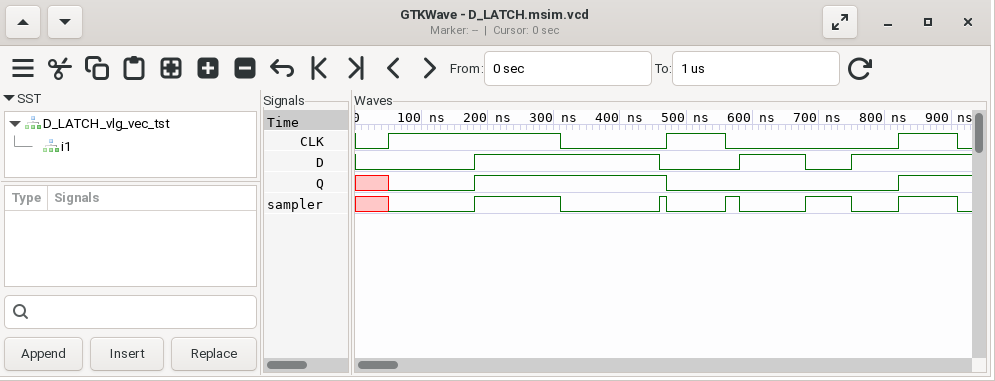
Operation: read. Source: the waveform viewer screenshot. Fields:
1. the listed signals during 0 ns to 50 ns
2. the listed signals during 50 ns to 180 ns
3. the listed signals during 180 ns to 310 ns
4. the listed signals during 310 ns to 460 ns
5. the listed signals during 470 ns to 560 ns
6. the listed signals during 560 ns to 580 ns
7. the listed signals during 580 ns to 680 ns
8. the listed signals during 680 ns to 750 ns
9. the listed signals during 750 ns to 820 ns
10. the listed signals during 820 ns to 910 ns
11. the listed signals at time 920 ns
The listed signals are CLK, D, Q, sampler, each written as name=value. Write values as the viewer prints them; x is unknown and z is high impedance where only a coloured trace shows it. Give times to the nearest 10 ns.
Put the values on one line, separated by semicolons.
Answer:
CLK=0, D=0, Q=x, sampler=x; CLK=1, D=0, Q=0, sampler=0; CLK=1, D=1, Q=1, sampler=1; CLK=0, D=1, Q=1, sampler=0; CLK=1, D=0, Q=0, sampler=0; CLK=0, D=0, Q=0, sampler=1; CLK=0, D=1, Q=0, sampler=0; CLK=0, D=0, Q=0, sampler=1; CLK=0, D=1, Q=0, sampler=0; CLK=1, D=1, Q=1, sampler=1; CLK=0, D=1, Q=1, sampler=0
